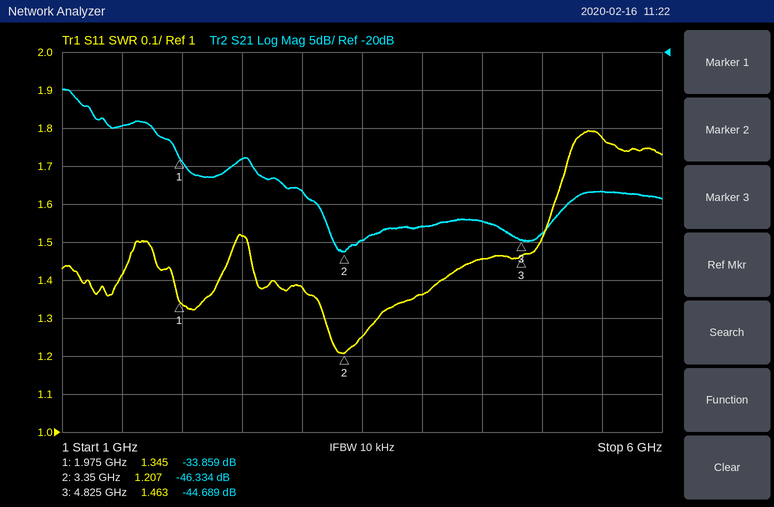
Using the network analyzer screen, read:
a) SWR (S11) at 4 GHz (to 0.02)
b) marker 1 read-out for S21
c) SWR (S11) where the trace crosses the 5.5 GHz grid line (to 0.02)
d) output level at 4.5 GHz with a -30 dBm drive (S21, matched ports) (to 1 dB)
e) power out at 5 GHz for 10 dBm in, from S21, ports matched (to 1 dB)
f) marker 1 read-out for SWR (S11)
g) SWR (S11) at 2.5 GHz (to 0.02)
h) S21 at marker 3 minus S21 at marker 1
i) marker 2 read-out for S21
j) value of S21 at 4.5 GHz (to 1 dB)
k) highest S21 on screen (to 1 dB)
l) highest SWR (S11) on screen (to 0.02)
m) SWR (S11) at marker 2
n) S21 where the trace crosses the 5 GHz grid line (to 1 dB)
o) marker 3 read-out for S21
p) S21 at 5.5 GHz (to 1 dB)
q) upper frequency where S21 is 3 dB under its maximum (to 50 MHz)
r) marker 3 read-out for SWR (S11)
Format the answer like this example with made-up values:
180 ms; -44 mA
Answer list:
1.36; -33.859 dB; 1.78; -72 dBm; -34 dBm; 1.345; 1.52; -10.830 dB; -46.334 dB; -42 dB; -25 dB; 1.80; 1.207; -44 dB; -44.689 dB; -38 dB; 1.25 GHz; 1.463
